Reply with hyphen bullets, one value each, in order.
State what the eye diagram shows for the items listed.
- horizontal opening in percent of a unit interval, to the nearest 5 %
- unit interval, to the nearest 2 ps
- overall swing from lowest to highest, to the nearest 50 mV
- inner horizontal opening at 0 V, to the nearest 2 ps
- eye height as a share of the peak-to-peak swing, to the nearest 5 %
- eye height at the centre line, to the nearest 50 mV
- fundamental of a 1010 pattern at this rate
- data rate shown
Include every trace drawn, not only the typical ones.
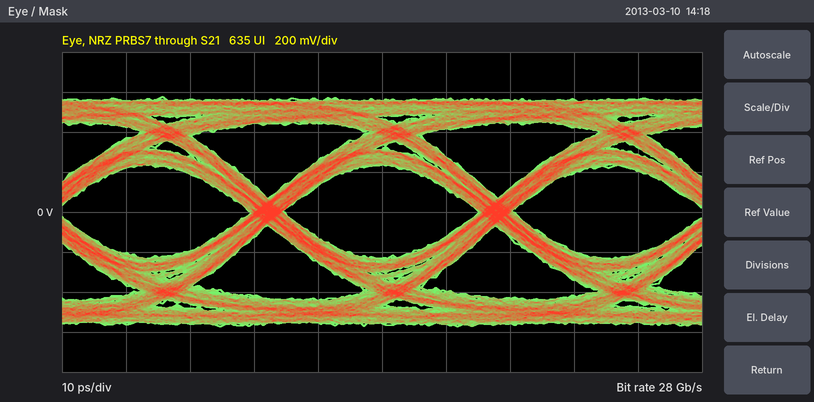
- 85 %
- 36 ps
- 1.15 V
- 30 ps
- 40 %
- 450 mV
- 14 GHz
- 28 Gb/s
